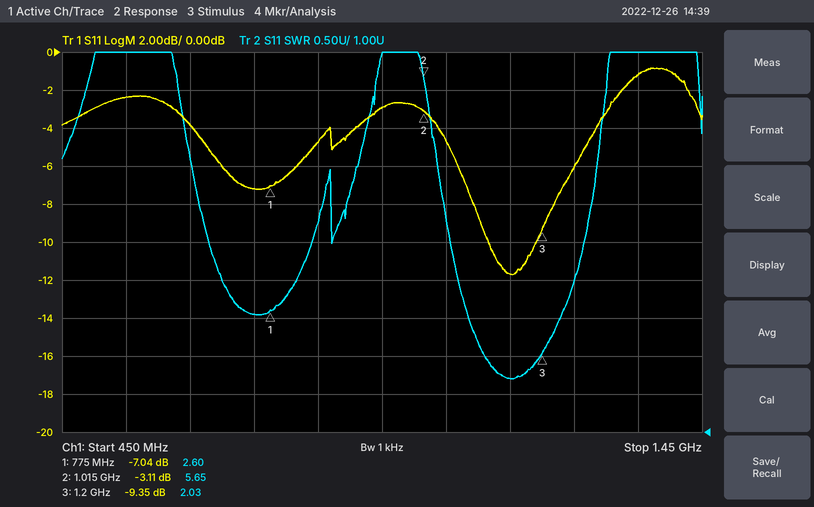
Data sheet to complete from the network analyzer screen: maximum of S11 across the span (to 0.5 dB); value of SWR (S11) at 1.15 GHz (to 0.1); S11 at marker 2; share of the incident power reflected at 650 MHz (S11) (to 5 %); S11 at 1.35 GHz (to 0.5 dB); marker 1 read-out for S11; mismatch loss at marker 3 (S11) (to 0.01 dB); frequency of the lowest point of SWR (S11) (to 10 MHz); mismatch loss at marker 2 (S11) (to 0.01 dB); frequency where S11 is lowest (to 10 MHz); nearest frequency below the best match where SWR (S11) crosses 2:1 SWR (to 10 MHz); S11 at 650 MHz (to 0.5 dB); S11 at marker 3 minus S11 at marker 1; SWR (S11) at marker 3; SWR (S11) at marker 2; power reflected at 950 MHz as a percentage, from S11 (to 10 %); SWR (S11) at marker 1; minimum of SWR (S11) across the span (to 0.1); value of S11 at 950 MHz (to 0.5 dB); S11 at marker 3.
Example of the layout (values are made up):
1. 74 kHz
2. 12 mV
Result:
1. -1.0 dB
2. 1.7
3. -3.11 dB
4. 40 %
5. -1.0 dB
6. -7.04 dB
7. 0.54 dB
8. 1.15 GHz
9. 2.91 dB
10. 1.15 GHz
11. 1.11 GHz
12. -4.0 dB
13. -2.31 dB
14. 2.03
15. 5.65
16. 50 %
17. 2.60
18. 1.7
19. -3.0 dB
20. -9.35 dB
